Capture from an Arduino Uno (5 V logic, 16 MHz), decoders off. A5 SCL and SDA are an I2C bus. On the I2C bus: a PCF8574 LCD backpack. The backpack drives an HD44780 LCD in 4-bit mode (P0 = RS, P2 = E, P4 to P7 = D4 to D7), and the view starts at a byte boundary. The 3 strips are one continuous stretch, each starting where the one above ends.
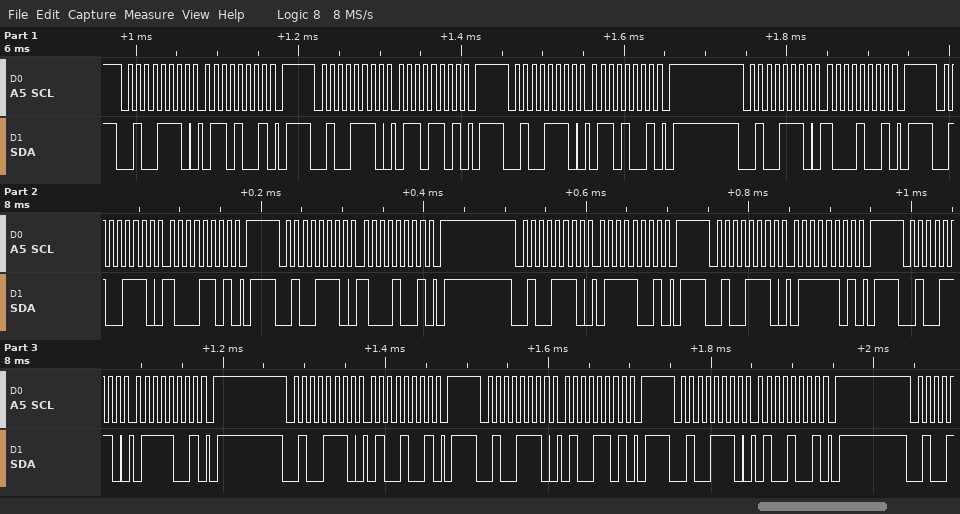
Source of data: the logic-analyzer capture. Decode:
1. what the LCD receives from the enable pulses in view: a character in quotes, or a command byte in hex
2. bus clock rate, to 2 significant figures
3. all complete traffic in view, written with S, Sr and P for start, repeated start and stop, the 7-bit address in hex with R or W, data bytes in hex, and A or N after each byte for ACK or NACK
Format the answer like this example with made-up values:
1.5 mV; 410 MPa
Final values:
'h' 't'; 100 kHz; S 27W A 69 A P S 27W A 6D A P S 27W A 69 A P S 27W A 89 A P S 27W A 8D A P S 27W A 89 A P S 27W A 79 A P S 27W A 7D A P S 27W A 79 A P S 27W A 49 A P S 27W A 4D A P S 27W A 49 A P
